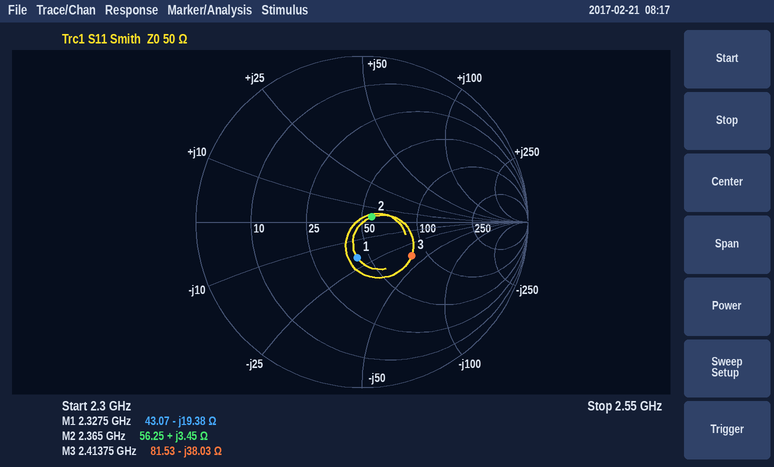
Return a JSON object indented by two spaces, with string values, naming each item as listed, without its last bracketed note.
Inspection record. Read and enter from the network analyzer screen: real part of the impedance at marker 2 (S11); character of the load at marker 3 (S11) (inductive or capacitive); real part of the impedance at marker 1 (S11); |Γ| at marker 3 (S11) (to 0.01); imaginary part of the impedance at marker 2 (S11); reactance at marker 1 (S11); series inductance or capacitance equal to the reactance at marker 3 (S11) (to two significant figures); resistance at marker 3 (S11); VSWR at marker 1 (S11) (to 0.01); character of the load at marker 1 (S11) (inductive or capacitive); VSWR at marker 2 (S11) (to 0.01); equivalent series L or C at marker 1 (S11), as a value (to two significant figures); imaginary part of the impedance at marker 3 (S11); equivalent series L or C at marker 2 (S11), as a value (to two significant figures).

{
  "real part of the impedance at marker 2": "56.25 Ω",
  "character of the load at marker 3 (S11)": "capacitive",
  "real part of the impedance at marker 1": "43.07 Ω",
  "|Γ| at marker 3 (S11)": "0.36",
  "imaginary part of the impedance at marker 2": "+3.45 Ω",
  "reactance at marker 1": "-19.38 Ω",
  "series inductance or capacitance equal to the reactance at marker 3 (S11)": "1.7 pF",
  "resistance at marker 3": "81.53 Ω",
  "VSWR at marker 1 (S11)": "1.55",
  "character of the load at marker 1 (S11)": "capacitive",
  "VSWR at marker 2 (S11)": "1.14",
  "equivalent series L or C at marker 1 (S11), as a value": "3.5 pF",
  "imaginary part of the impedance at marker 3": "-38.03 Ω",
  "equivalent series L or C at marker 2 (S11), as a value": "230 pH"
}
